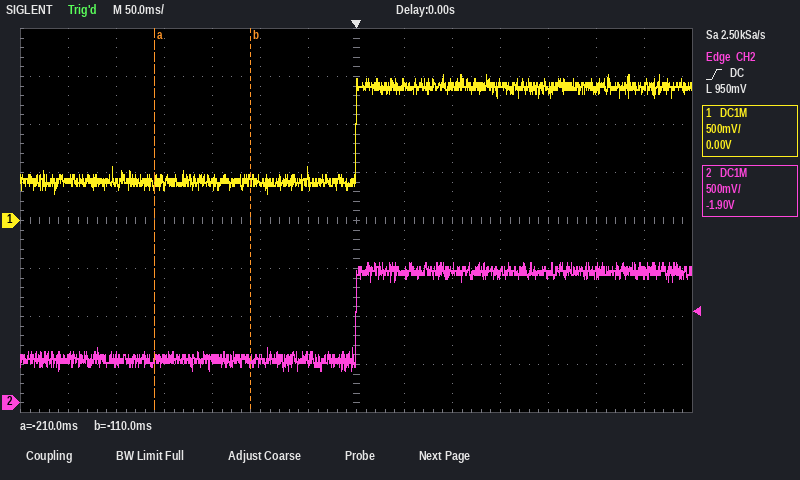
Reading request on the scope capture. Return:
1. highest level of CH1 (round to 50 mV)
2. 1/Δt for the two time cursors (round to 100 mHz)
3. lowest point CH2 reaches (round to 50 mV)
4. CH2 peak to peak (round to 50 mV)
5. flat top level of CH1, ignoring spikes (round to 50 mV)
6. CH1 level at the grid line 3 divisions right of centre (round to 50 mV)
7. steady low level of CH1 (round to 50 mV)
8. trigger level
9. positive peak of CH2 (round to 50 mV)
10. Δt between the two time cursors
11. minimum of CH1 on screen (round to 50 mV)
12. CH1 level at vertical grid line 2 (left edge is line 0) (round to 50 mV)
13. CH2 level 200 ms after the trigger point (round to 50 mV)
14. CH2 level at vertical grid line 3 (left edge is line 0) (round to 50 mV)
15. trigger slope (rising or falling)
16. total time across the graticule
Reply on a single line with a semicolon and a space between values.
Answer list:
1.50 V; 10.0 Hz; 350 mV; 1.10 V; 1.40 V; 1.45 V; 400 mV; 950 mV; 1.45 V; 100 ms; 300 mV; 400 mV; 1.35 V; 450 mV; rising; 700 ms
